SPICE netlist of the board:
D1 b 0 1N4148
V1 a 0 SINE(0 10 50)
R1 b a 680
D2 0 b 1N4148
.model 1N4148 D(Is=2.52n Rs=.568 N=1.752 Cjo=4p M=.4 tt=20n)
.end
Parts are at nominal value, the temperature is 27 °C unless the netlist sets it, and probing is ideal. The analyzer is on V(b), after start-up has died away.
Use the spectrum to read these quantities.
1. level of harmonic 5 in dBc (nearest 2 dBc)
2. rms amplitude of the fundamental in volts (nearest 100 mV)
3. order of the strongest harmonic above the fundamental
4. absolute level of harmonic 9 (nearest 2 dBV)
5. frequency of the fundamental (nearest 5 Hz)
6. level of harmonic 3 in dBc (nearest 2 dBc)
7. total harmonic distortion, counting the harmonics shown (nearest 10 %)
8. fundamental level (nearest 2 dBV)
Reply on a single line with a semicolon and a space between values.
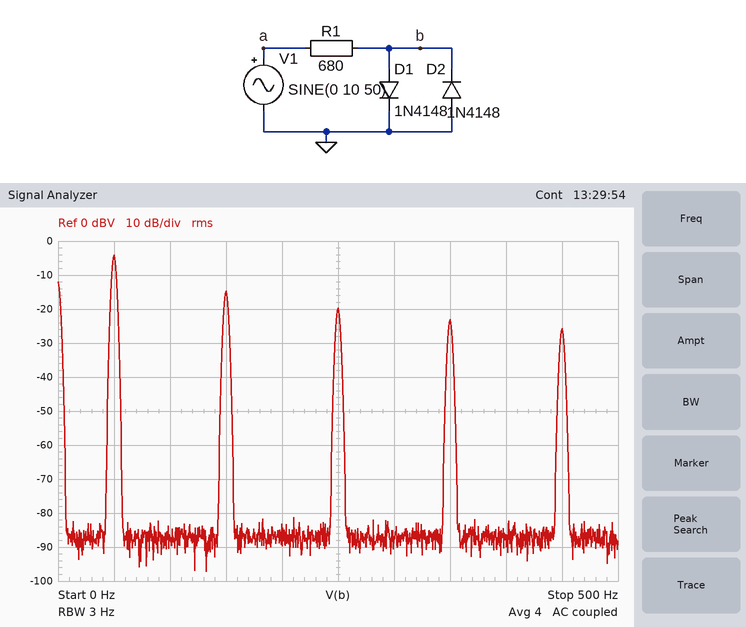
-16 dBc; 600 mV; 3; -26 dBV; 50 Hz; -10 dBc; 40 %; -4 dBV
